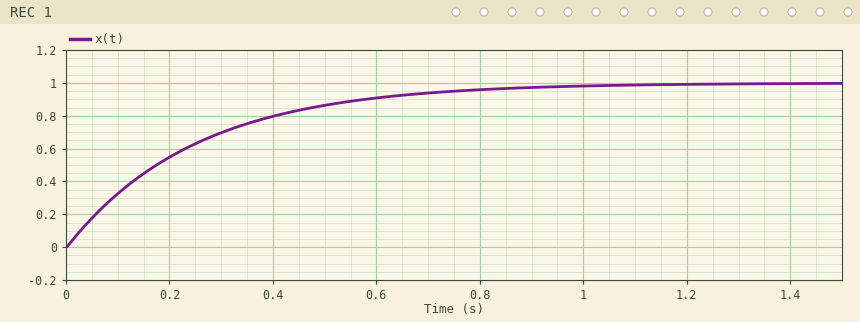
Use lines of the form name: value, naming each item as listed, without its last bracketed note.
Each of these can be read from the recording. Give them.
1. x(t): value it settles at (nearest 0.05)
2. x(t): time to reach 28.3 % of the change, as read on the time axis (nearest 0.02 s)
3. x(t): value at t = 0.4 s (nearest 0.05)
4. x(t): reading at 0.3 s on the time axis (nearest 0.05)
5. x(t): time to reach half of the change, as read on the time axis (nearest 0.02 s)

x(t): value it settles at: 1.00
x(t): time to reach 28.3 % of the change, as read on the time axis: 0.08 s
x(t): value at t = 0.4 s: 0.80
x(t): reading at 0.3 s on the time axis: 0.70
x(t): time to reach half of the change, as read on the time axis: 0.18 s
